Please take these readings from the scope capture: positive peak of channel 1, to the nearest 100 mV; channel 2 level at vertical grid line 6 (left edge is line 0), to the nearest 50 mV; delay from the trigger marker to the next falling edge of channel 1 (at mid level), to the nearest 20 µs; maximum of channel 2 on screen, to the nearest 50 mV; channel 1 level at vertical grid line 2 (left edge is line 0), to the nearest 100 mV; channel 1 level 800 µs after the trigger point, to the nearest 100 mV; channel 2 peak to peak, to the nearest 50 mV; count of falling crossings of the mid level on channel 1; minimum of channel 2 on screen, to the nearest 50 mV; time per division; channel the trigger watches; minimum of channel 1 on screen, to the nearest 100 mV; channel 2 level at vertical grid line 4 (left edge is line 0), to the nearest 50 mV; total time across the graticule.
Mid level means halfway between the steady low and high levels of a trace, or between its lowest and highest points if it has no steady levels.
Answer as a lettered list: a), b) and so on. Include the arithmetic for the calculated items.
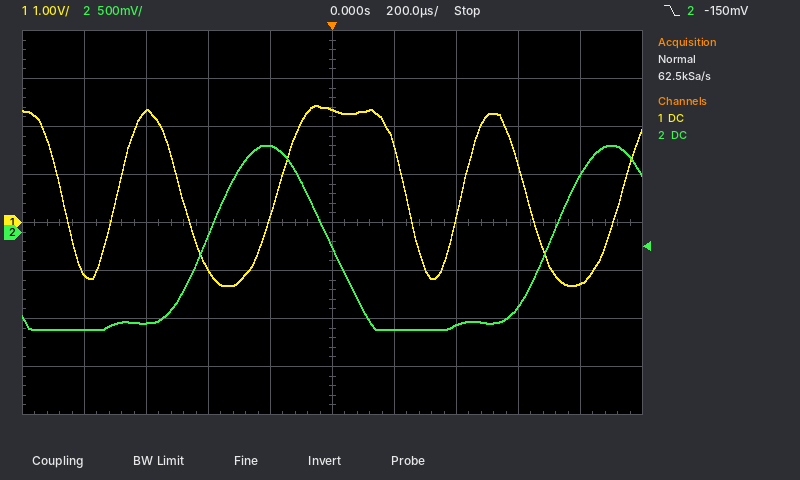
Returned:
a) 2.4 V
b) -1.00 V
c) 240 µs
d) 900 mV
e) 2.3 V
f) -1.3 V
g) 900 mV − (-1.00 V) = 1.90 V
h) 4
i) -1.00 V
j) 200 µs
k) channel 2
l) -1.3 V
m) 900 mV
n) 2 ms
